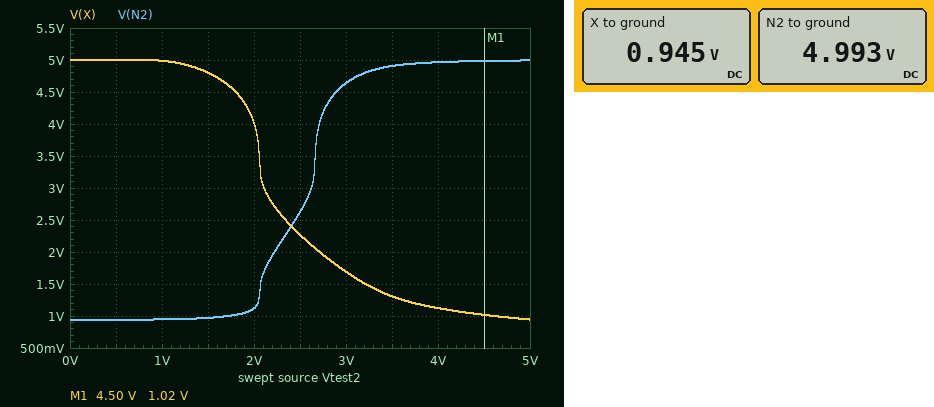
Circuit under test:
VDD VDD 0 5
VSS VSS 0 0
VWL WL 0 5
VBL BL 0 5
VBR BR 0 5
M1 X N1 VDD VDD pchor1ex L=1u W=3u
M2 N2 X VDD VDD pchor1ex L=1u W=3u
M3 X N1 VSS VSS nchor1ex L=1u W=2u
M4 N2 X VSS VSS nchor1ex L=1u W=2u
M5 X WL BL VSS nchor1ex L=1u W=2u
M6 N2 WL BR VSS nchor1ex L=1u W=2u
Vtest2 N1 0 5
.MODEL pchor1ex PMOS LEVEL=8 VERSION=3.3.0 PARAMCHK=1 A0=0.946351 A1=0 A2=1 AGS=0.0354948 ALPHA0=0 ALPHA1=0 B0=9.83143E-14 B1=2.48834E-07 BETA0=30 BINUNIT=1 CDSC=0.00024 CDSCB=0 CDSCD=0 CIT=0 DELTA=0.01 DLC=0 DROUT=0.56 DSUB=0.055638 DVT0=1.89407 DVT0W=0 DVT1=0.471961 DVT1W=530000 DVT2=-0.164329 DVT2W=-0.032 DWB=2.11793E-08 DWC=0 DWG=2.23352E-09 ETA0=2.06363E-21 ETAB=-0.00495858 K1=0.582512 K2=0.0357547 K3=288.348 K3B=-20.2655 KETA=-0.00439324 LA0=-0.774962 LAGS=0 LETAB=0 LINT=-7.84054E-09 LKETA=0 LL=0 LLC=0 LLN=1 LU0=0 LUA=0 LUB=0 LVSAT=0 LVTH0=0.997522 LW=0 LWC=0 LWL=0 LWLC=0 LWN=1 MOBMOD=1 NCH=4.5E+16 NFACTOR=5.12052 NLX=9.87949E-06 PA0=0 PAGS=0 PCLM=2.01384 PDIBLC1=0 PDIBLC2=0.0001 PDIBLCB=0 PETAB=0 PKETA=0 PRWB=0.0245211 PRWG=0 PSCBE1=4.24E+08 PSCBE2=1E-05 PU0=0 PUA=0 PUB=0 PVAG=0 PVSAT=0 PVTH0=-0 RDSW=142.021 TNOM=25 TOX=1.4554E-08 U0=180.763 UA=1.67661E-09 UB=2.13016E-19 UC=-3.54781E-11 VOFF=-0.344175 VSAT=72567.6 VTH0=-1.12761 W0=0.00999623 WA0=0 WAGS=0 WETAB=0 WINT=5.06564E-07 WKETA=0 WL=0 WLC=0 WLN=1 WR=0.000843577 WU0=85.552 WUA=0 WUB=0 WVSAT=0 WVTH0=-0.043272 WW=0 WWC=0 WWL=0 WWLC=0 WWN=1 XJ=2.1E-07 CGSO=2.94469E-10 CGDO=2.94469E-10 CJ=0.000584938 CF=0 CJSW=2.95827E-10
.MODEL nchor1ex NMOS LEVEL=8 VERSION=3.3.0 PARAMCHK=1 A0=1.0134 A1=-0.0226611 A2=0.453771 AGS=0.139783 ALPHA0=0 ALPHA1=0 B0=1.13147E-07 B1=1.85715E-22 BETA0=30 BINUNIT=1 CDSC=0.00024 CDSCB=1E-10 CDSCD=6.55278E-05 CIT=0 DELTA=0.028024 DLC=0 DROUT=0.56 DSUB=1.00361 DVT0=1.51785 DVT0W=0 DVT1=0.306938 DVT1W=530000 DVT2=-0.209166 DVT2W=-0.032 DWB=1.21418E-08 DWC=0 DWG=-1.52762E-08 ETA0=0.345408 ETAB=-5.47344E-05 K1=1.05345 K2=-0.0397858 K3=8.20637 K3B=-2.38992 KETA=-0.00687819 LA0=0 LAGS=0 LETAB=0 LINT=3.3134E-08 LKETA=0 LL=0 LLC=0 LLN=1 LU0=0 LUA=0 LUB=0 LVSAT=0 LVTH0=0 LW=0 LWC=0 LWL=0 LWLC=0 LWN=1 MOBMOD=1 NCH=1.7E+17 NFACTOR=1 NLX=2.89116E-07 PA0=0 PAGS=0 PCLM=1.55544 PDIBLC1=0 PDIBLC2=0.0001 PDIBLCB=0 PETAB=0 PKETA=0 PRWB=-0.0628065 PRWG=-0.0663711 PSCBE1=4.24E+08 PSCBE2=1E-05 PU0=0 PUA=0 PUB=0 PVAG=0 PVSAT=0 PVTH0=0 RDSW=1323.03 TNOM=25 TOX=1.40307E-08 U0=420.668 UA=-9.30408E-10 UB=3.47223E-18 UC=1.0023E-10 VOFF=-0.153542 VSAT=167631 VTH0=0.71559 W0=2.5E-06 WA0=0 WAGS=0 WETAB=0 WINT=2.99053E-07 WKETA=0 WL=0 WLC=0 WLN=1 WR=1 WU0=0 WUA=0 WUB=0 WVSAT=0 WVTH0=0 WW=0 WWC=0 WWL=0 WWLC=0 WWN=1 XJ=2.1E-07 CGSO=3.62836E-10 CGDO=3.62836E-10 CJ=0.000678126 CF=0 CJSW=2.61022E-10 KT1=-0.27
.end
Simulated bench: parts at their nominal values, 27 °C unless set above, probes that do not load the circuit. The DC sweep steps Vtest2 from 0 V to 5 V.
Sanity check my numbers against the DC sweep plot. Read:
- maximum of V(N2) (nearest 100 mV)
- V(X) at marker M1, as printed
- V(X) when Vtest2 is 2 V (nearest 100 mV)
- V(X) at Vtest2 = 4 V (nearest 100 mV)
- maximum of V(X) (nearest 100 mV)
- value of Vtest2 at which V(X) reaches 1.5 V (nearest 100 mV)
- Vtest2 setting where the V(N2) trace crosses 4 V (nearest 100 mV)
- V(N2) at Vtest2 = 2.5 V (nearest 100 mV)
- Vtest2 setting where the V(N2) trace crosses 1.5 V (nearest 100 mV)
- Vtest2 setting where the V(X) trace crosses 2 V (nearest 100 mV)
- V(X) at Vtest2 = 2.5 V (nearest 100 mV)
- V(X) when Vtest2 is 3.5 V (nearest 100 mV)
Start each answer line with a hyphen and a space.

- 5.0 V
- 1.02 V
- 4.0 V
- 1.1 V
- 5.0 V
- 3.2 V
- 2.7 V
- 2.6 V
- 2.1 V
- 2.7 V
- 2.3 V
- 1.3 V
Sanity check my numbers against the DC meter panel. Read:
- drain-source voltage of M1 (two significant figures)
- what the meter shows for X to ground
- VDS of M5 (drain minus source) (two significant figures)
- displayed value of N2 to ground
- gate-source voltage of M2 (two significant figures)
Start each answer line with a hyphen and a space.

- -4.1 V
- 0.945 V
- -4.1 V
- 4.993 V
- -4.1 V
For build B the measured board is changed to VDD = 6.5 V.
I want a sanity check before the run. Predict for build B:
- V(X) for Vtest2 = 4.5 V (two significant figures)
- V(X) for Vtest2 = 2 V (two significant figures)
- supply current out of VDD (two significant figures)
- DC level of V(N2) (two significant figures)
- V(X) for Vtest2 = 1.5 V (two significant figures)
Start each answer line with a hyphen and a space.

- 1.1 V
- 6.1 V
- 3.6 µA
- 6.5 V
- 6.4 V
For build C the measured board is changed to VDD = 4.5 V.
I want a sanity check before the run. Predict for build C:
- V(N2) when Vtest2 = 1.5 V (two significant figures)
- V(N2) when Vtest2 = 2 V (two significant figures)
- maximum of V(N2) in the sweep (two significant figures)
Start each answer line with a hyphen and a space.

- 1.1 V
- 1.8 V
- 4.5 V
